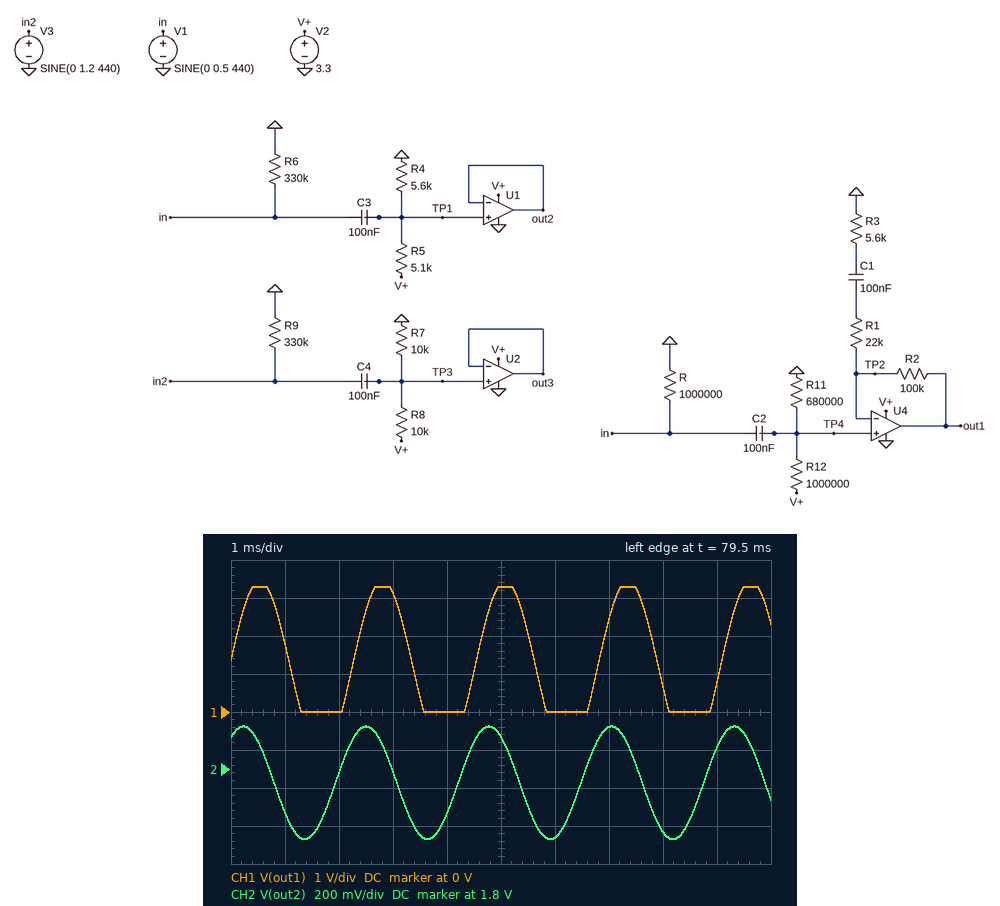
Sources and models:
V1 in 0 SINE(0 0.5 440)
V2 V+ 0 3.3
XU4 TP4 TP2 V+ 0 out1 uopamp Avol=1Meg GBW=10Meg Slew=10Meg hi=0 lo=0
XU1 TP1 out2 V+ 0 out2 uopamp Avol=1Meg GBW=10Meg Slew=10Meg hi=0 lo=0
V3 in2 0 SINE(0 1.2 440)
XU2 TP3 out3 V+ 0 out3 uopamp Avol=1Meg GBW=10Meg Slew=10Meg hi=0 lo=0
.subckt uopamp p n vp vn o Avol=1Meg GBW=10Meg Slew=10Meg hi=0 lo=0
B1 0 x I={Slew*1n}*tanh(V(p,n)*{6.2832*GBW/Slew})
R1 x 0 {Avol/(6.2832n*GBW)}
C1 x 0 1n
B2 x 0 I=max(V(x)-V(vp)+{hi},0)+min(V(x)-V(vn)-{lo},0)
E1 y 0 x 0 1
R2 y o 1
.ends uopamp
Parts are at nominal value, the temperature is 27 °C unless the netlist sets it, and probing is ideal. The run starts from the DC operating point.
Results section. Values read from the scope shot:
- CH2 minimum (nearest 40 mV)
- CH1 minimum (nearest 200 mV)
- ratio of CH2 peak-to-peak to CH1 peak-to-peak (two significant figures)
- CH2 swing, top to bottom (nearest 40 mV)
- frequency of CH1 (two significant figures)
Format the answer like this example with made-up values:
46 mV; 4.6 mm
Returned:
1.44 V; 0 V; 0.18; 600 mV; 440 Hz
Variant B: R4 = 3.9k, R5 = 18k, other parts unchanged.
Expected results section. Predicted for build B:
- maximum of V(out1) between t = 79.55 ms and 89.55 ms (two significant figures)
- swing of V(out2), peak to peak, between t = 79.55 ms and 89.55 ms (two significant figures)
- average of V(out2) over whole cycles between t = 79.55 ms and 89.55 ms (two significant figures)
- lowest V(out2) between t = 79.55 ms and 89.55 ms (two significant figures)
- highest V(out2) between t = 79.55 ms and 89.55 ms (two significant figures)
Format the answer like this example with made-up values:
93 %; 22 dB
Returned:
3.3 V; 660 mV; 590 mV; 260 mV; 920 mV
